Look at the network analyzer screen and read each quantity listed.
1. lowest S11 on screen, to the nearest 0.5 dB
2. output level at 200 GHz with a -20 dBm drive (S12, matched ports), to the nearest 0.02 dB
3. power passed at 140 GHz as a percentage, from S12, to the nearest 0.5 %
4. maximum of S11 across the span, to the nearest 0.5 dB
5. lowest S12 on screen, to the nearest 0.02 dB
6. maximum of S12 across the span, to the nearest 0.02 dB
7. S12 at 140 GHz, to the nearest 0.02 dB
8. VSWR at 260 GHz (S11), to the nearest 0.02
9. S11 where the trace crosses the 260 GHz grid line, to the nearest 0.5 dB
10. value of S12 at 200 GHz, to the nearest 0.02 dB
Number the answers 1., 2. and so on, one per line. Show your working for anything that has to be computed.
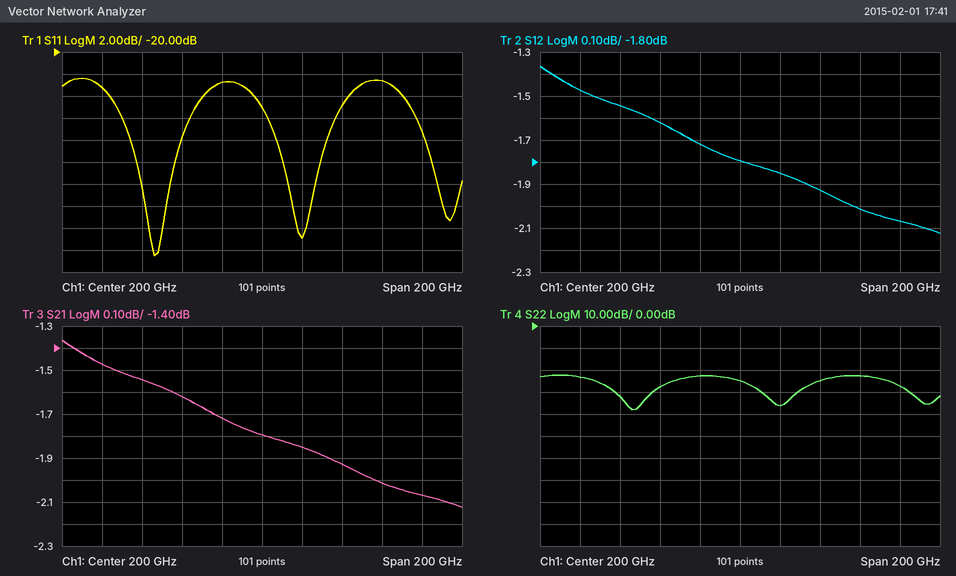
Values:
1. -38.5 dB
2. -20 dBm + (-1.80 dB) = -21.80 dBm
3. 10^(-1.54/10) ≈ 70.1 %, so 70.0 % to the nearest 0.5 %
4. -22.5 dB
5. -2.12 dB
6. -1.36 dB
7. -1.54 dB
8. |Γ| = 10^(-22.5/20) = 0.0750; VSWR = (1 + 0.0750)/(1 − 0.0750) ≈ 1.16
9. -22.5 dB
10. -1.80 dB
